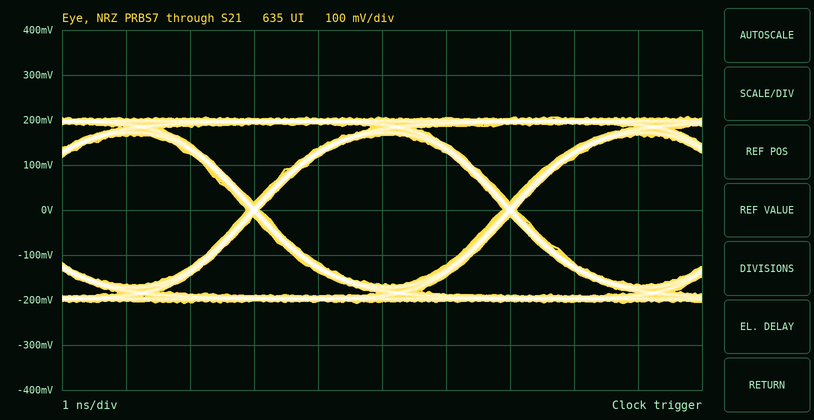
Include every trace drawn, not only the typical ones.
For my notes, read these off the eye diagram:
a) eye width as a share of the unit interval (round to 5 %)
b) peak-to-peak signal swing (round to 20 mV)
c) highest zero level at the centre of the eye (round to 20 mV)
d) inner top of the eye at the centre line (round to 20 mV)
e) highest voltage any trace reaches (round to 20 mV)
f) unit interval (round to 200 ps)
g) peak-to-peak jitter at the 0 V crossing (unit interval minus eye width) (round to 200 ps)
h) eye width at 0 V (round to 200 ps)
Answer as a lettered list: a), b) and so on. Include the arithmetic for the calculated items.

a) 3.8 ns / 4.0 ns ≈ 95 %
b) 420 mV
c) -160 mV
d) 160 mV
e) 200 mV
f) 4.0 ns
g) 200 ps
h) 3.8 ns
